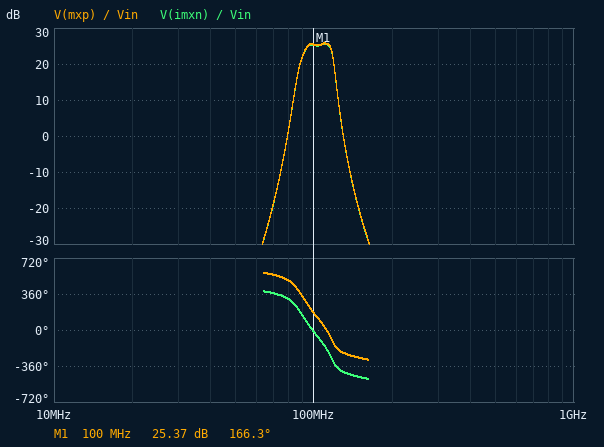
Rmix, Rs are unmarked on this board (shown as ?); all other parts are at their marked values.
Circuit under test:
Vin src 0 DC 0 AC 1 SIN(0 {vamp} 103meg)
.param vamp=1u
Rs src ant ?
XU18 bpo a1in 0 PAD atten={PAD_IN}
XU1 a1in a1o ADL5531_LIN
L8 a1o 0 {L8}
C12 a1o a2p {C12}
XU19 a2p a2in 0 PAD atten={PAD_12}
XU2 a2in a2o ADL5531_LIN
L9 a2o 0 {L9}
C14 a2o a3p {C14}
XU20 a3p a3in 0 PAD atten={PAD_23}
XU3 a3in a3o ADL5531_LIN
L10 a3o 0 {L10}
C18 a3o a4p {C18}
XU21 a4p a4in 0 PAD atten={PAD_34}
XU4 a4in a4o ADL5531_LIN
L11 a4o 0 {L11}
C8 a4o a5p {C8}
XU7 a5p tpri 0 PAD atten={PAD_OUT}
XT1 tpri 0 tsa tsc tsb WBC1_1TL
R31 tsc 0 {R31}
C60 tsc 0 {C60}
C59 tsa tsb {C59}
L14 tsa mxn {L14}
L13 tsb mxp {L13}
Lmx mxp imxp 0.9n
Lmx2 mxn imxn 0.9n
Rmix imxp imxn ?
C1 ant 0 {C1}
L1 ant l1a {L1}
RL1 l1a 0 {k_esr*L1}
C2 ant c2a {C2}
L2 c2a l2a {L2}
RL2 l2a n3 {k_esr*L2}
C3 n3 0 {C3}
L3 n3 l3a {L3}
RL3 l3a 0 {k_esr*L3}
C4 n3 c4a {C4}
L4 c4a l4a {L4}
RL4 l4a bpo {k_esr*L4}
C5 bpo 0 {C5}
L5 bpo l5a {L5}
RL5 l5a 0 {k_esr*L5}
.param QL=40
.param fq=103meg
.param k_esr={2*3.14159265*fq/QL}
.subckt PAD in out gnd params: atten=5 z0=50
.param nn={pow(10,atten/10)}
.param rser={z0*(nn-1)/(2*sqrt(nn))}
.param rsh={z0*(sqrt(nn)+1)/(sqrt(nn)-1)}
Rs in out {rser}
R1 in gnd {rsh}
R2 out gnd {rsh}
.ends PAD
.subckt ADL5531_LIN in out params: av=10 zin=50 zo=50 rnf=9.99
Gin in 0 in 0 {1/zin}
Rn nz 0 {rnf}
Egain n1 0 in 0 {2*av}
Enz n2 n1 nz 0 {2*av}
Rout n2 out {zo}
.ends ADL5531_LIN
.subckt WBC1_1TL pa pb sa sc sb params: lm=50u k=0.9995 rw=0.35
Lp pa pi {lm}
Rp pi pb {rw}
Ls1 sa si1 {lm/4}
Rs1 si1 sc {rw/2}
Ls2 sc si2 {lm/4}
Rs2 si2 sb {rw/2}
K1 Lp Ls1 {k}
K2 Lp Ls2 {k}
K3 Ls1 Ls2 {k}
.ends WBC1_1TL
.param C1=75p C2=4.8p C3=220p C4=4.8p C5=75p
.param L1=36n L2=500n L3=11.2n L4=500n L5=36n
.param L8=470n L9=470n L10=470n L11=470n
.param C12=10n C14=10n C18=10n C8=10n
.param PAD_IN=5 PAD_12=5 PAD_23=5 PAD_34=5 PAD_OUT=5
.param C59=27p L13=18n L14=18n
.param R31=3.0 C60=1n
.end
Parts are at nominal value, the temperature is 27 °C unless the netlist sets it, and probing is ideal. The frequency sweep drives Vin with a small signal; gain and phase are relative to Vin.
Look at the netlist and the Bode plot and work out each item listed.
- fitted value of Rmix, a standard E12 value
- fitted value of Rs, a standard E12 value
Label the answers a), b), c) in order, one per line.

a) 8.2 Ω
b) 100 Ω
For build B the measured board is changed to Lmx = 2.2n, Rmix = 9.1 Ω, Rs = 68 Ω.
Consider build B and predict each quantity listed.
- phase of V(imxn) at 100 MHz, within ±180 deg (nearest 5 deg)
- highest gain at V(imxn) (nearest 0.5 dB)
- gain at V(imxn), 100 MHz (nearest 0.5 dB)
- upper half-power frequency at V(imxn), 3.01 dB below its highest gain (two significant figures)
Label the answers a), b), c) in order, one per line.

a) -15 deg
b) 28.5 dB
c) 28.0 dB
d) 120 MHz
